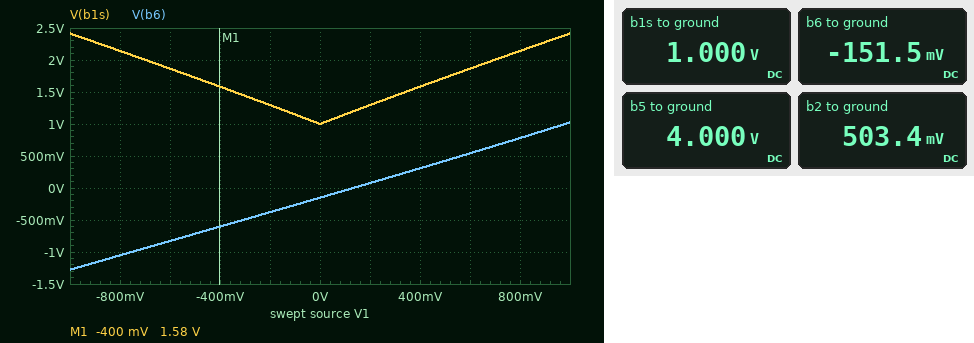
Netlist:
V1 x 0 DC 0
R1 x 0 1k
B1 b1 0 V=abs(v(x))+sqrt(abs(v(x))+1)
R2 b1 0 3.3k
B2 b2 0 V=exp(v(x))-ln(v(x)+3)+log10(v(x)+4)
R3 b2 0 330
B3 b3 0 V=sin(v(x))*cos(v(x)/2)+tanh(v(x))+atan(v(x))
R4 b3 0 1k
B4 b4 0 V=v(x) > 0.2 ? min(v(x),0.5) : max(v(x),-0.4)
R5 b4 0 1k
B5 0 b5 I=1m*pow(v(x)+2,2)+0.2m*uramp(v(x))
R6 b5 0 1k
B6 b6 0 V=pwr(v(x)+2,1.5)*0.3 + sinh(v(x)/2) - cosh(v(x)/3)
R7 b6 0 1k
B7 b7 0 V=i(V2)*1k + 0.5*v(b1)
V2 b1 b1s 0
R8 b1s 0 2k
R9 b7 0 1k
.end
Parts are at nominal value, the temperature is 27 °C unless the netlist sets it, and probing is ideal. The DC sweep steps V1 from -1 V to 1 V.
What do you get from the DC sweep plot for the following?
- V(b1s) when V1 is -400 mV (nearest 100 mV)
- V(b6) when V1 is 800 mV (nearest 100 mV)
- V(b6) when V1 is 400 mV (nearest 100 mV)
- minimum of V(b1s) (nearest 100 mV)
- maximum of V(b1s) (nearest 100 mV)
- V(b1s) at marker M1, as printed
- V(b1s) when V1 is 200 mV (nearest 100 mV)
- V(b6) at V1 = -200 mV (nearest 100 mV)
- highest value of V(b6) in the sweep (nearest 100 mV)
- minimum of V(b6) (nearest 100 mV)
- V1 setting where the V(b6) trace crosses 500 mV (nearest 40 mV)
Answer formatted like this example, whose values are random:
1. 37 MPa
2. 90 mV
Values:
1. 1.6 V
2. 800 mV
3. 300 mV
4. 1.0 V
5. 2.4 V
6. 1.58 V
7. 1.3 V
8. -400 mV
9. 1.0 V
10. -1.3 V
11. 560 mV
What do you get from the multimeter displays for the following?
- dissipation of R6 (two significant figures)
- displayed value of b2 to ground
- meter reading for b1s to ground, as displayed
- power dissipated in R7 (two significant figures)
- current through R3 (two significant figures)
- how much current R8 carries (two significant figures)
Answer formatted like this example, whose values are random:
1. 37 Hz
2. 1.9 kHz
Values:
1. 16 mW
2. 503.4 mV
3. 1.000 V
4. 23 µW
5. 1.5 mA
6. 500 µA
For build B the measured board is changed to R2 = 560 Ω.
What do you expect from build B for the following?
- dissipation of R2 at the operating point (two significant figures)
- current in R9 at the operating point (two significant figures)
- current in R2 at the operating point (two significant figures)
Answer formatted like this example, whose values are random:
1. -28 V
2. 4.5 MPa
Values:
1. 1.8 mW
2. 1.0 mA
3. 1.8 mA
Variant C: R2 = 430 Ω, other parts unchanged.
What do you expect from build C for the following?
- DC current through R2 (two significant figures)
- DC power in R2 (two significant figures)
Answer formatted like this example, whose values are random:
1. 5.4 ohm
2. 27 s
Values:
1. 2.3 mA
2. 2.3 mW
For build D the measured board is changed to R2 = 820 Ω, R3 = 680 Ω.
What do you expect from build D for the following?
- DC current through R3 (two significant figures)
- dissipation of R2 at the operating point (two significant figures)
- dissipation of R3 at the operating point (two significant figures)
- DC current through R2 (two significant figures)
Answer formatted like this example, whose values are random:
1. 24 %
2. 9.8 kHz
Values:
1. 740 µA
2. 1.2 mW
3. 370 µW
4. 1.2 mA
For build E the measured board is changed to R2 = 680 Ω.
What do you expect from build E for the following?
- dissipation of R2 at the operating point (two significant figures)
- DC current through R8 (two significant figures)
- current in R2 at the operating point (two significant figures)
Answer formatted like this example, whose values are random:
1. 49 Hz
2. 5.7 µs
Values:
1. 1.5 mW
2. 500 µA
3. 1.5 mA
